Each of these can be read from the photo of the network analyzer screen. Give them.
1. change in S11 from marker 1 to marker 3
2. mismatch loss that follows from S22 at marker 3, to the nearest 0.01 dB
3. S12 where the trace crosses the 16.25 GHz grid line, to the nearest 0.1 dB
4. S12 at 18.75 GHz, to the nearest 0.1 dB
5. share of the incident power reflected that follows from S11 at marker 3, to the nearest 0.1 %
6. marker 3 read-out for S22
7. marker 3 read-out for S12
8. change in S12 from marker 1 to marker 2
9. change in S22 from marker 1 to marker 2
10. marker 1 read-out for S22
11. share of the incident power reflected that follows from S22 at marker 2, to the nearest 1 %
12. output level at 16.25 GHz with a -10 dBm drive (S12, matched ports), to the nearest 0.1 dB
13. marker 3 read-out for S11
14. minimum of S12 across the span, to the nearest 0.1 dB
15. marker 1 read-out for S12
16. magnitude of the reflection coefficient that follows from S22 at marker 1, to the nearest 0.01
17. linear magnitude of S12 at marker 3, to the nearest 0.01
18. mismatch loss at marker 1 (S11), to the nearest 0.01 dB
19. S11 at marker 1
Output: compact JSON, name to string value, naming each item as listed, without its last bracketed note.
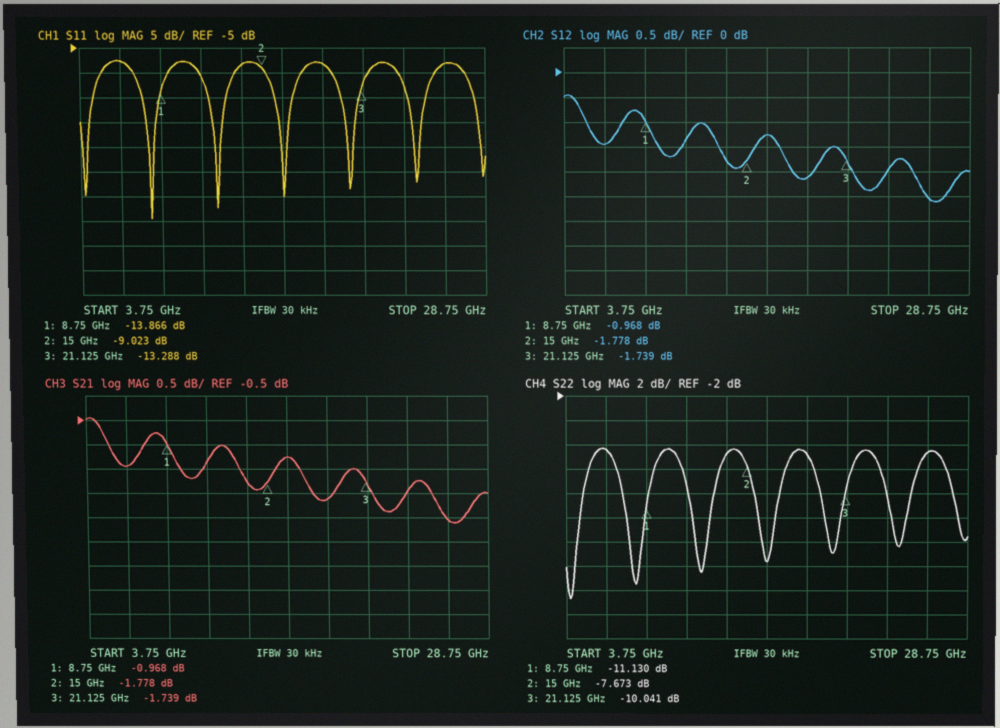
{"change in S11 from marker 1 to marker 3": "0.578 dB", "mismatch loss that follows from S22 at marker 3, to the nearest 0.01 dB": "0.45 dB", "S12 where the trace crosses the 16.25 GHz grid line, to the nearest 0.1 dB": "-1.3 dB", "S12 at 18.75 GHz, to the nearest 0.1 dB": "-2.1 dB", "share of the incident power reflected that follows from S11 at marker 3, to the nearest 0.1 %": "4.7 %", "marker 3 read-out for S22": "-10.041 dB", "marker 3 read-out for S12": "-1.739 dB", "change in S12 from marker 1 to marker 2": "-0.810 dB", "change in S22 from marker 1 to marker 2": "3.457 dB", "marker 1 read-out for S22": "-11.130 dB", "share of the incident power reflected that follows from S22 at marker 2, to the nearest 1 %": "17 %", "output level at 16.25 GHz with a -10 dBm drive (S12, matched ports), to the nearest 0.1 dB": "-11.3 dBm", "marker 3 read-out for S11": "-13.288 dB", "minimum of S12 across the span, to the nearest 0.1 dB": "-2.6 dB", "marker 1 read-out for S12": "-0.968 dB", "magnitude of the reflection coefficient that follows from S22 at marker 1, to the nearest 0.01": "0.28", "linear magnitude of S12 at marker 3, to the nearest 0.01": "0.82", "mismatch loss at marker 1 (S11), to the nearest 0.01 dB": "0.18 dB", "S11 at marker 1": "-13.866 dB"}
